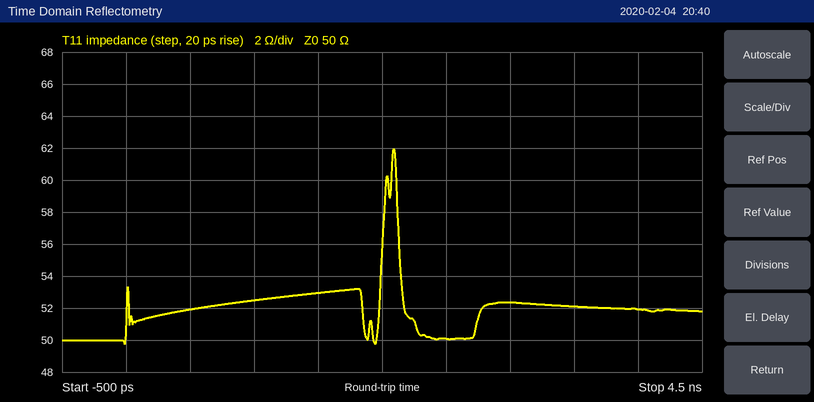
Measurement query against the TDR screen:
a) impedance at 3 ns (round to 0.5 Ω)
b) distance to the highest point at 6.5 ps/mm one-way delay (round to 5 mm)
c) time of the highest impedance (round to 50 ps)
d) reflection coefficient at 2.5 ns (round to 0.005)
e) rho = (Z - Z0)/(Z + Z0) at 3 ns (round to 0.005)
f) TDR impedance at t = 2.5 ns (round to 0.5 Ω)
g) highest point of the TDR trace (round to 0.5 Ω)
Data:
52.5 Ω
160 mm
2.10 ns
0.000
+0.025
50.0 Ω
62.0 Ω
